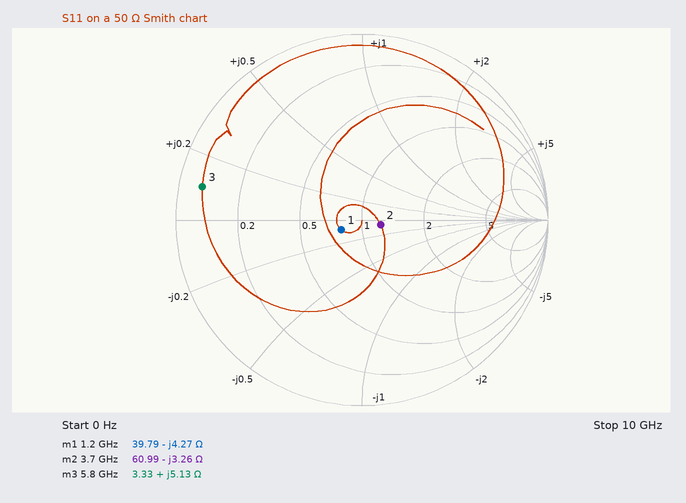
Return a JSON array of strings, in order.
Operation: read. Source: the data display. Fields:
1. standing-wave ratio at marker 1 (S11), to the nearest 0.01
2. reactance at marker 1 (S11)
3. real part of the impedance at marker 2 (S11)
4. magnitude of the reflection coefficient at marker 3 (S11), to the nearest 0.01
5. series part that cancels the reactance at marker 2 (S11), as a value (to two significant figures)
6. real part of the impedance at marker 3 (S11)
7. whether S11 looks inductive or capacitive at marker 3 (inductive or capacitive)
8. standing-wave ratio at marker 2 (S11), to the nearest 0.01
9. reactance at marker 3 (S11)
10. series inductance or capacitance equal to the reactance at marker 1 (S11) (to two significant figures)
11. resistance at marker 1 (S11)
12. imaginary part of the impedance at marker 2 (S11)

["1.28", "-4.27 Ω", "60.99 Ω", "0.88", "140 pH", "3.33 Ω", "inductive", "1.23", "+5.13 Ω", "31 pF", "39.79 Ω", "-3.26 Ω"]
